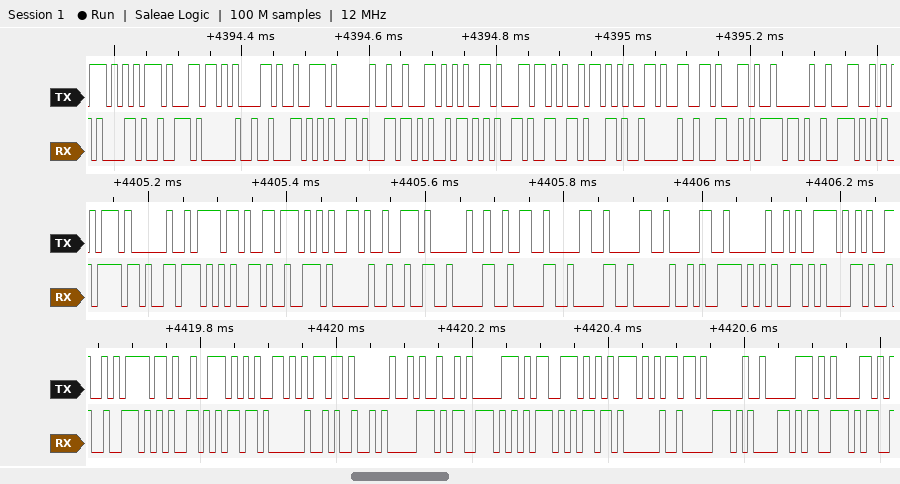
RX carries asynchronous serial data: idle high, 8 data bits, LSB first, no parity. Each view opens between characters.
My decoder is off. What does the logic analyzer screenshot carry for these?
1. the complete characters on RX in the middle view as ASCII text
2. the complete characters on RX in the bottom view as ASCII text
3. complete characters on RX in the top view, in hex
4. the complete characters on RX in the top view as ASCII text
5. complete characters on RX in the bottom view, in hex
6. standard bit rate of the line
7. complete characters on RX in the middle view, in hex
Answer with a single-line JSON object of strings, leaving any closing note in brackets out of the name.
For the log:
{"the complete characters on RX in the middle view as ASCII text": "\"over 2000 yea\"", "the complete characters on RX in the bottom view as ASCII text": "\"rem Ipsum pas\"", "complete characters on RX in the top view, in hex": "61, 72, 20, 62, 65, 6C, 69, 65, 66, 2C, 20, 4C, 6F, 72", "the complete characters on RX in the top view as ASCII text": "\"ar belief, Lor\"", "complete characters on RX in the bottom view, in hex": "72, 65, 6D, 20, 49, 70, 73, 75, 6D, 20, 70, 61, 73", "standard bit rate of the line": "115200 baud", "complete characters on RX in the middle view, in hex": "6F, 76, 65, 72, 20, 32, 30, 30, 30, 20, 79, 65, 61"}
